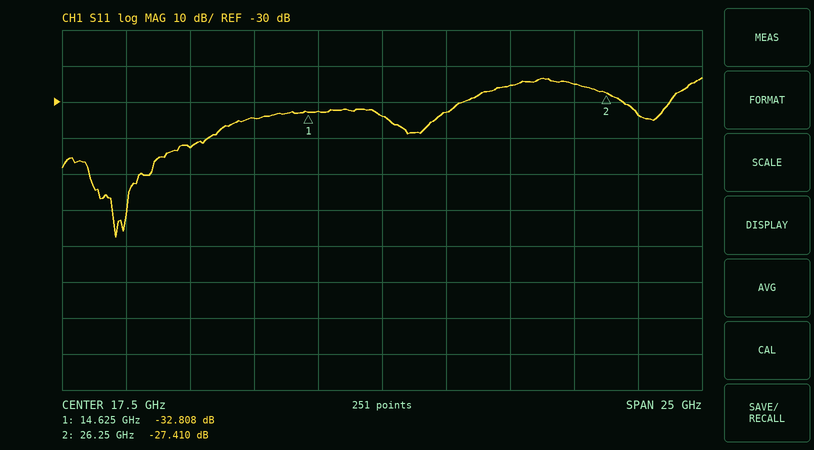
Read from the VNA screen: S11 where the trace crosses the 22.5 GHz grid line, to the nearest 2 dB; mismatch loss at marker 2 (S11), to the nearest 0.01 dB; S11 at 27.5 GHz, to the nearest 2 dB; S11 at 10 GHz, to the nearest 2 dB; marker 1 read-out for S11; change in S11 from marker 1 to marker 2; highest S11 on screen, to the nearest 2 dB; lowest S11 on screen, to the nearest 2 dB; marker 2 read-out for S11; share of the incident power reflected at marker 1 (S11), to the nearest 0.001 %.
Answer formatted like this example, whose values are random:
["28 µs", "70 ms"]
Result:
["-26 dB", "0.01 dB", "-34 dB", "-42 dB", "-32.808 dB", "5.398 dB", "-24 dB", "-68 dB", "-27.410 dB", "0.052 %"]
